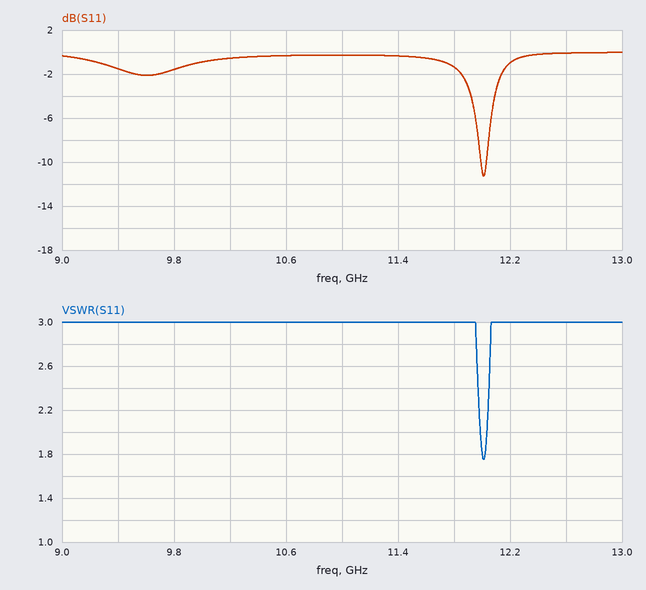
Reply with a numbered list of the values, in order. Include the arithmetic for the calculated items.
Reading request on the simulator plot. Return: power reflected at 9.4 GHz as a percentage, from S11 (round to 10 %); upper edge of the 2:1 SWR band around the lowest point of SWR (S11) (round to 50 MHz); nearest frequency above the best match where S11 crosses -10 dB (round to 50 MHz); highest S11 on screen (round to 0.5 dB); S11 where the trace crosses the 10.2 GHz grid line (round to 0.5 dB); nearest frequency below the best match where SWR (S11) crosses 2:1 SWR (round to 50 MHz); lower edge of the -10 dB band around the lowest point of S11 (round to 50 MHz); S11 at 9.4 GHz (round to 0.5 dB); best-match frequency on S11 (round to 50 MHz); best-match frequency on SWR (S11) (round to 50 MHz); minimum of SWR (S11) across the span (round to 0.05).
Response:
1. 10^(-1.5/10) ≈ 70.8 %, so 70 % to the nearest 10 %
2. 12.05 GHz
3. 12.05 GHz
4. 0.0 dB
5. -0.5 dB
6. 12.00 GHz
7. 12.00 GHz
8. -1.5 dB
9. 12.00 GHz
10. 12.00 GHz
11. 1.75
